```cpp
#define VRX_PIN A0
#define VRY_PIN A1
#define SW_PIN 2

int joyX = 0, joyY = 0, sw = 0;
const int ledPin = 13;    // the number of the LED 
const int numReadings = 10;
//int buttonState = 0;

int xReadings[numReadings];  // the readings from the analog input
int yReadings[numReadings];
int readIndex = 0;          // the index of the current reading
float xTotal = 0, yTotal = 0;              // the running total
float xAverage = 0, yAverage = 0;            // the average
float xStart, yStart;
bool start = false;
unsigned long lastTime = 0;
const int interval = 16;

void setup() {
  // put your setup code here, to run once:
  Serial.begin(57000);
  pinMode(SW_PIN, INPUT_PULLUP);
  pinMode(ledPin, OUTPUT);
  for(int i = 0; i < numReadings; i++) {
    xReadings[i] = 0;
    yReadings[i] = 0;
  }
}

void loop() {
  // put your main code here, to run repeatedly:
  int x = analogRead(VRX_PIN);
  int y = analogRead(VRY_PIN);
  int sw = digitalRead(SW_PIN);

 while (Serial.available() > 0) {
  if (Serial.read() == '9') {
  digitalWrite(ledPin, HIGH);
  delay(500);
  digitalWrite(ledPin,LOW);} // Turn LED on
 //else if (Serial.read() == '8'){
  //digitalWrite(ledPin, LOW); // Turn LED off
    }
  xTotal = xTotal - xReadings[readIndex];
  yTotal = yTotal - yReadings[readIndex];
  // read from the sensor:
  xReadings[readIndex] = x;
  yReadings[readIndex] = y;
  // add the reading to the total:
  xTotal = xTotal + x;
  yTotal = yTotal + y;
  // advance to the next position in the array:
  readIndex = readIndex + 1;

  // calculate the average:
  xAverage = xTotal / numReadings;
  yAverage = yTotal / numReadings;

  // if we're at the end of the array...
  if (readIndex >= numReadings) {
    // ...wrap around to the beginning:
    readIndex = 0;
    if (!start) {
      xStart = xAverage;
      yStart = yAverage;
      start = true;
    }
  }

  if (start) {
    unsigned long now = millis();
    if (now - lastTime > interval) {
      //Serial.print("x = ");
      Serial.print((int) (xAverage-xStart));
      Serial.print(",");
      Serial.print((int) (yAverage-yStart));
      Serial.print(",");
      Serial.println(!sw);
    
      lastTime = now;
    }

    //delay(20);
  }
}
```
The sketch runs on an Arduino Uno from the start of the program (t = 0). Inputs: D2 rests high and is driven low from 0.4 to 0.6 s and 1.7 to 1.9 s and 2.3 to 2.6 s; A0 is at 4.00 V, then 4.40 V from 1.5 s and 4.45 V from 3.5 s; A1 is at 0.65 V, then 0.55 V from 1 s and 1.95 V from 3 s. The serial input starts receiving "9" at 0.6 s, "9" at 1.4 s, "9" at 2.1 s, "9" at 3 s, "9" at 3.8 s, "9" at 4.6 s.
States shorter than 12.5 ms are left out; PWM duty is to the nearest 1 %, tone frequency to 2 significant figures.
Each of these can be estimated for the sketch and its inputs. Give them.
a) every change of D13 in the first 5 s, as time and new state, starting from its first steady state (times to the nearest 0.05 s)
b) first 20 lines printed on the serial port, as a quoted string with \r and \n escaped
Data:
0 s low; 0.6 s high; 1.1 s low; 1.4 s high; 1.9 s low; 2.1 s high; 2.6 s low; 3 s high; 3.5 s low; 3.8 s high; 4.3 s low; 4.6 s high
"0,0,0\r\n0,0,0\r\n0,0,0\r\n0,0,0\r\n0,0,0\r\n0,0,0\r\n0,0,0\r\n0,0,0\r\n0,0,0\r\n0,0,0\r\n0,0,0\r\n0,0,0\r\n0,0,0\r\n0,0,0\r\n0,0,0\r\n0,0,0\r\n0,0,0\r\n0,0,0\r\n0,0,0\r\n0,0,0\r\n"
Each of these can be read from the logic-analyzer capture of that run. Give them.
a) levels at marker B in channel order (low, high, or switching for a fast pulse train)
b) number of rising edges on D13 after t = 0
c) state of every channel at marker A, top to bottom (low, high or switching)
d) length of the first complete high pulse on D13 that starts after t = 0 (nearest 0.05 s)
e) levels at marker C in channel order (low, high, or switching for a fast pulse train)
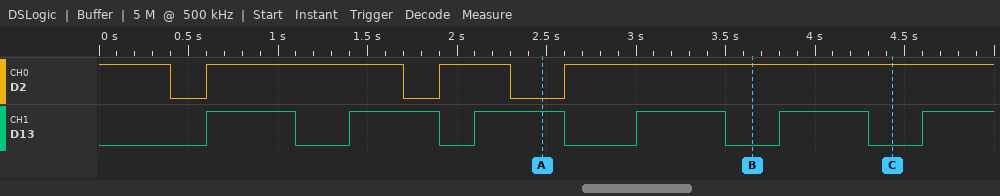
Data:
D2 high, D13 low
6
D2 low, D13 high
0.50 s
D2 high, D13 low
